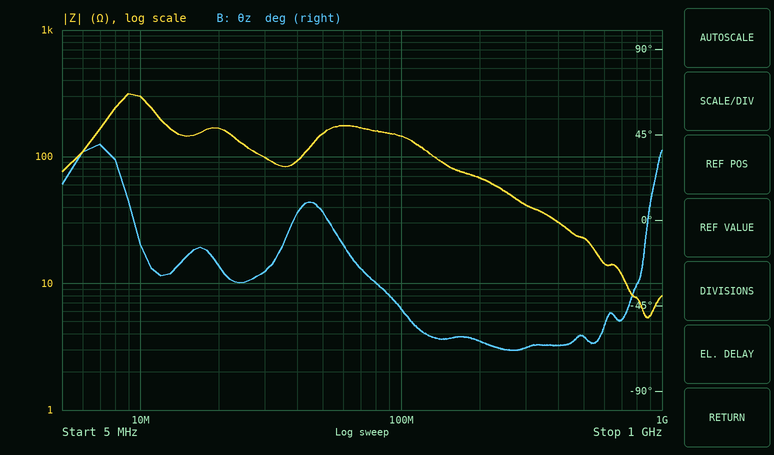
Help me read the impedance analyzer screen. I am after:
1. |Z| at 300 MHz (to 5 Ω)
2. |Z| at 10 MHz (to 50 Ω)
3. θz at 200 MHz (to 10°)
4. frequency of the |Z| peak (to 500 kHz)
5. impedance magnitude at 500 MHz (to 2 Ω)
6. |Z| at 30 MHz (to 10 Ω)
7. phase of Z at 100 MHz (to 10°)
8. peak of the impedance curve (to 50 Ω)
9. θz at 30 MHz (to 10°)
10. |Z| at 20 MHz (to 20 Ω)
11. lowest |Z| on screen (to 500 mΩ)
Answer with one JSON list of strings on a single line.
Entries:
["40 Ω", "300 Ω", "-60°", "9.0 MHz", "22 Ω", "100 Ω", "-50°", "300 Ω", "-30°", "160 Ω", "5.5 Ω"]
